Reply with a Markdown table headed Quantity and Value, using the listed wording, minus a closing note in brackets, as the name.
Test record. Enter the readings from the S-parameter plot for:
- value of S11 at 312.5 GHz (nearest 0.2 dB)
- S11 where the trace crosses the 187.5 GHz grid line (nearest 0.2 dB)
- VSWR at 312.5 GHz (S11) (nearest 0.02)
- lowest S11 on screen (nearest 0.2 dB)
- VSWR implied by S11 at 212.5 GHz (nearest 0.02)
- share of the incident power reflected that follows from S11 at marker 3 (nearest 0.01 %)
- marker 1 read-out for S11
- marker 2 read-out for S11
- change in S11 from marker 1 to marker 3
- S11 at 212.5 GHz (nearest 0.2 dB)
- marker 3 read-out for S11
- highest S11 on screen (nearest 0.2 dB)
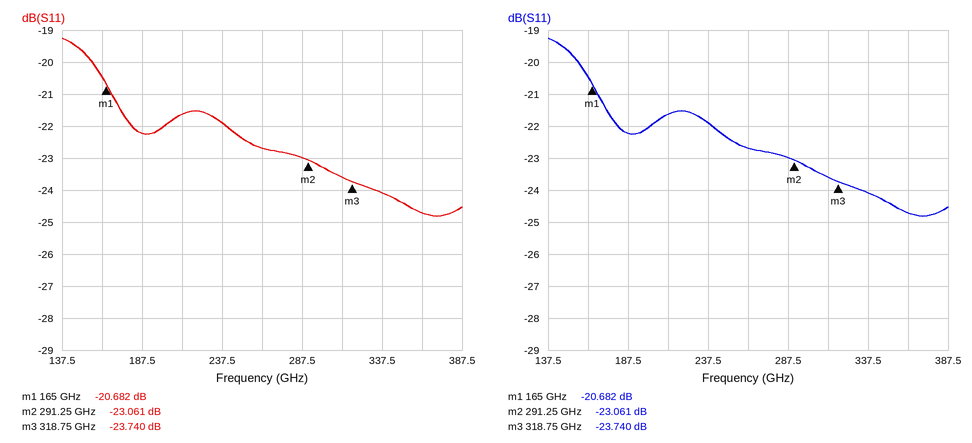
| Quantity | Value |
|---|---|
| value of S11 at 312.5 GHz | -23.6 dB |
| S11 where the trace crosses the 187.5 GHz grid line | -22.2 dB |
| VSWR at 312.5 GHz (S11) | 1.14 |
| lowest S11 on screen | -24.8 dB |
| VSWR implied by S11 at 212.5 GHz | 1.18 |
| share of the incident power reflected that follows from S11 at marker 3 | 0.42 % |
| marker 1 read-out for S11 | -20.682 dB |
| marker 2 read-out for S11 | -23.061 dB |
| change in S11 from marker 1 to marker 3 | -3.058 dB |
| S11 at 212.5 GHz | -21.6 dB |
| marker 3 read-out for S11 | -23.740 dB |
| highest S11 on screen | -19.2 dB |
